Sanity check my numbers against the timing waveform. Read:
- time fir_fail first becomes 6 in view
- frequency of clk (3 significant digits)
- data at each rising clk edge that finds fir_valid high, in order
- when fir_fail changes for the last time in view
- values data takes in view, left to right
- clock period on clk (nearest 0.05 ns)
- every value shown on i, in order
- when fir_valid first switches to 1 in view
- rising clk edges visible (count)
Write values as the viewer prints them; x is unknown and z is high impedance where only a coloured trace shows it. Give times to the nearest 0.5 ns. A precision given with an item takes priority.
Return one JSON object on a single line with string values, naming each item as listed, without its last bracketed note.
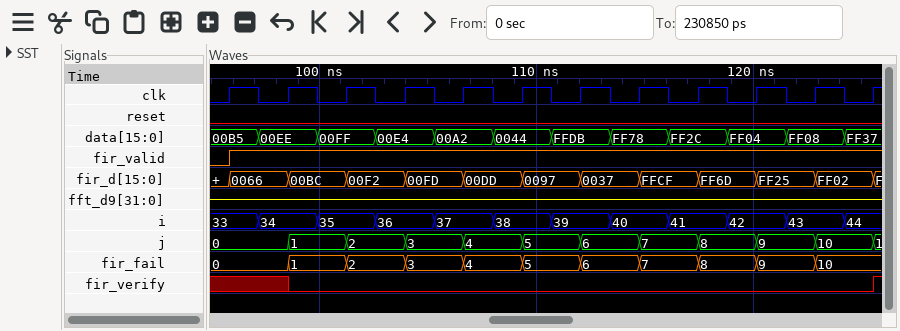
{"time fir_fail first becomes 6 in view": "112 ns", "frequency of clk": "370 MHz", "data at each rising clk edge that finds fir_valid high, in order": "00EE, 00FF, 00E4, 00A2, 0044, FFDB, FF78, FF2C, FF04, FF08, FF37", "when fir_fail changes for the last time in view": "123 ns", "values data takes in view, left to right": "00B5, 00EE, 00FF, 00E4, 00A2, 0044, FFDB, FF78, FF2C, FF04, FF08, FF37", "clock period on clk": "2.7 ns", "every value shown on i, in order": "33, 34, 35, 36, 37, 38, 39, 40, 41, 42, 43, 44", "when fir_valid first switches to 1 in view": "96 ns", "rising clk edges visible": "12"}
